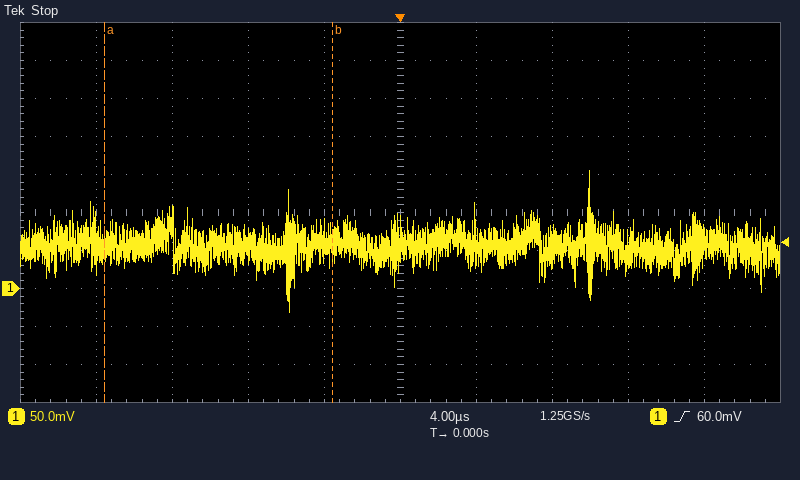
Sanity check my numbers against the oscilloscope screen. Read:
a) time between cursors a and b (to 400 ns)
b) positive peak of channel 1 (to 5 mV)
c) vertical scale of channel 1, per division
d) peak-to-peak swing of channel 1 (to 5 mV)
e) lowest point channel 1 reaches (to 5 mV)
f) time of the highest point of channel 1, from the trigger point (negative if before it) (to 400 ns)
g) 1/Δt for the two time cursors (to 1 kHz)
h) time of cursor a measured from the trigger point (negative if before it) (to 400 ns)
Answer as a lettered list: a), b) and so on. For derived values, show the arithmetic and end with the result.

a) 12.0 µs
b) 155 mV
c) 50 mV
d) 155 mV − (-30 mV) = 185 mV
e) -30 mV
f) +10.0 µs
g) 1 / 12.0 µs ≈ 83 kHz
h) -15.6 µs
